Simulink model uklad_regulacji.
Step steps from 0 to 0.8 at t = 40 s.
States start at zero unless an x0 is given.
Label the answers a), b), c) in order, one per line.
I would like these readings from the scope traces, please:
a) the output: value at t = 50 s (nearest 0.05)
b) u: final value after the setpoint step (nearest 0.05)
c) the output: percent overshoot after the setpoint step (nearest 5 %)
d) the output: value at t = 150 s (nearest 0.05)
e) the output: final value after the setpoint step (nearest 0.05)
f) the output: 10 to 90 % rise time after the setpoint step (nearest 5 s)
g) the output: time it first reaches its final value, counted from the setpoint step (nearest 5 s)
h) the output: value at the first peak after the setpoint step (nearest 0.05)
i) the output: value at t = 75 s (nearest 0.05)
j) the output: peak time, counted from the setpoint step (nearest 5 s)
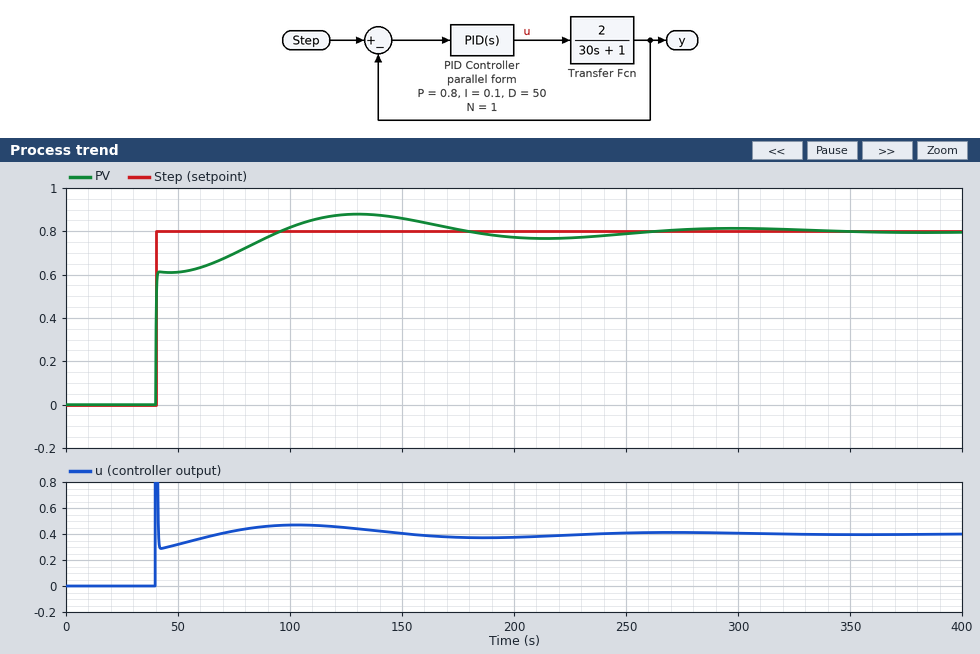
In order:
a) 0.60
b) 0.40
c) 10 %
d) 0.85
e) 0.80
f) 40 s
g) 55 s
h) 0.90
i) 0.70
j) 90 s
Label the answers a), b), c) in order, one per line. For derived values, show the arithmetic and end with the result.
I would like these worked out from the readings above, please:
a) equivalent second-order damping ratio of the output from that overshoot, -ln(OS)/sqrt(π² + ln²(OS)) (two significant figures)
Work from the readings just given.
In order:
a) ln(0.1) = -2.303; 2.303 / sqrt(9.870 + 5.302) = 0.59
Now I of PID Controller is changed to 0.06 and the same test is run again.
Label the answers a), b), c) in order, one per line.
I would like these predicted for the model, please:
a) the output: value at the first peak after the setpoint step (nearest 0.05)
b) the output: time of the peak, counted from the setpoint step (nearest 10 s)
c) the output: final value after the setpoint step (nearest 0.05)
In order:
a) 0.85
b) 120 s
c) 0.80
